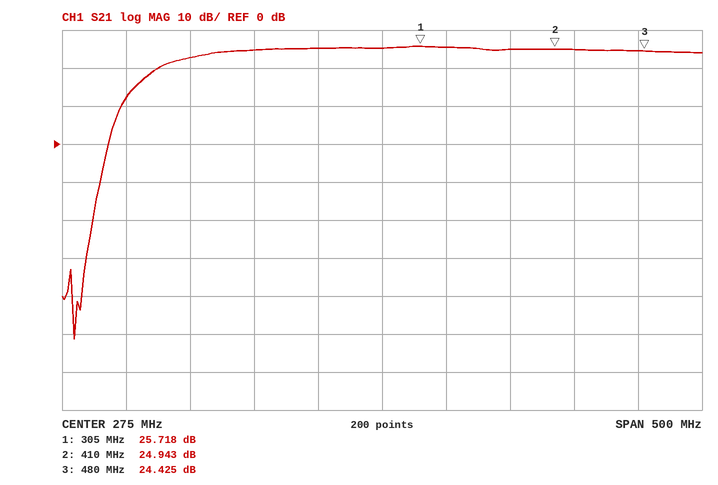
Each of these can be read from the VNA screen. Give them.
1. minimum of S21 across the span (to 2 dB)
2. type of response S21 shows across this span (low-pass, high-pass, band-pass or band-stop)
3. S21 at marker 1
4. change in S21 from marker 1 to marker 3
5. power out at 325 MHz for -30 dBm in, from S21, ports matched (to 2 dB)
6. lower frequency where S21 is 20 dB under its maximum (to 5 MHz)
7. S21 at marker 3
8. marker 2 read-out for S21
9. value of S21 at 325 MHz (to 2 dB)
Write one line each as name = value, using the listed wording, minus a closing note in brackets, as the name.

minimum of S21 across the span = -52 dB
type of response S21 shows across this span = high-pass
S21 at marker 1 = 25.718 dB
change in S21 from marker 1 to marker 3 = -1.293 dB
power out at 325 MHz for -30 dBm in, from S21, ports matched = -4 dBm
lower frequency where S21 is 20 dB under its maximum = 65 MHz
S21 at marker 3 = 24.425 dB
marker 2 read-out for S21 = 24.943 dB
value of S21 at 325 MHz = 26 dB
